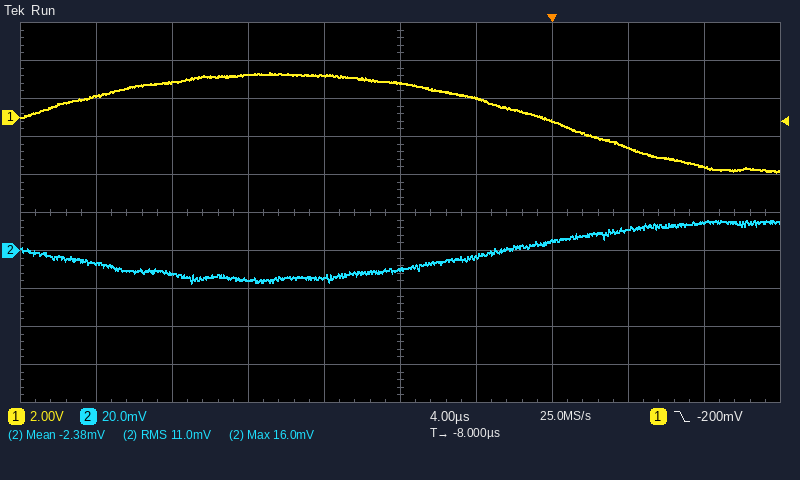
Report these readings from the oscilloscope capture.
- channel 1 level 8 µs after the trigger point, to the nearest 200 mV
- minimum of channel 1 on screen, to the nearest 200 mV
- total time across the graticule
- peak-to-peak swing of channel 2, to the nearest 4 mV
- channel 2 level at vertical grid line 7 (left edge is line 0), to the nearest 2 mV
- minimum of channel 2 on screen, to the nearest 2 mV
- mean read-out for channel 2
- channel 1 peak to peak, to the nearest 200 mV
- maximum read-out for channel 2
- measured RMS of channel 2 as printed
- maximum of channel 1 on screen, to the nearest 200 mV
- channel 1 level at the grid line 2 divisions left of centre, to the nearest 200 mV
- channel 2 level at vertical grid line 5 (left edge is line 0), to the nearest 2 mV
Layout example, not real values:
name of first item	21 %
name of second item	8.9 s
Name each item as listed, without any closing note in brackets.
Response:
channel 1 level 8 µs after the trigger point, to the nearest 200 mV	-2.6 V
minimum of channel 1 on screen, to the nearest 200 mV	-2.8 V
total time across the graticule	40 µs
peak-to-peak swing of channel 2, to the nearest 4 mV	32 mV
channel 2 level at vertical grid line 7 (left edge is line 0), to the nearest 2 mV	4 mV
minimum of channel 2 on screen, to the nearest 2 mV	-18 mV
mean read-out for channel 2	-2.38 mV
channel 1 peak to peak, to the nearest 200 mV	5.2 V
maximum read-out for channel 2	16.0 mV
measured RMS of channel 2 as printed	11.0 mV
maximum of channel 1 on screen, to the nearest 200 mV	2.4 V
channel 1 level at the grid line 2 divisions left of centre, to the nearest 200 mV	2.2 V
channel 2 level at vertical grid line 5 (left edge is line 0), to the nearest 2 mV	-10 mV
